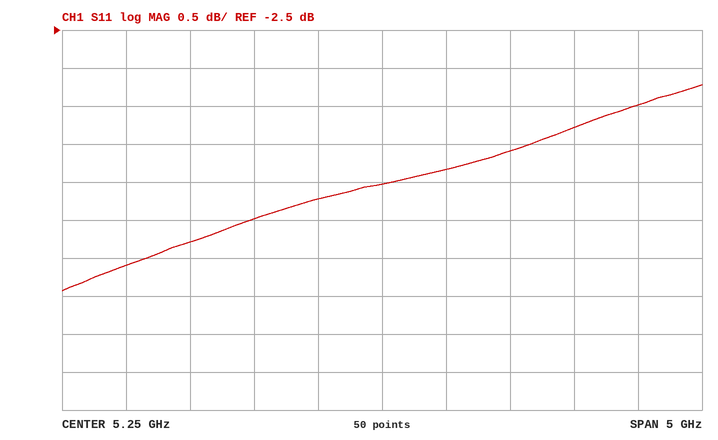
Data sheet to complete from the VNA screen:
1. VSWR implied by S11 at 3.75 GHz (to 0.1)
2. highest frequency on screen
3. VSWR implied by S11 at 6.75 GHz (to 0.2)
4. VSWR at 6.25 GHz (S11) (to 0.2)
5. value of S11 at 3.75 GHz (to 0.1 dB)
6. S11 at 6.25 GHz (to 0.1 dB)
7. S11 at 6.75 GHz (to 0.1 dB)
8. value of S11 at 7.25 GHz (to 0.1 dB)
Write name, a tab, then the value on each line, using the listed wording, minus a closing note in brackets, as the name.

VSWR implied by S11 at 3.75 GHz	3.4
highest frequency on screen	7.75 GHz
VSWR implied by S11 at 6.75 GHz	4.6
VSWR at 6.25 GHz (S11)	4.4
value of S11 at 3.75 GHz	-5.3 dB
S11 at 6.25 GHz	-4.1 dB
S11 at 6.75 GHz	-3.8 dB
value of S11 at 7.25 GHz	-3.5 dB
